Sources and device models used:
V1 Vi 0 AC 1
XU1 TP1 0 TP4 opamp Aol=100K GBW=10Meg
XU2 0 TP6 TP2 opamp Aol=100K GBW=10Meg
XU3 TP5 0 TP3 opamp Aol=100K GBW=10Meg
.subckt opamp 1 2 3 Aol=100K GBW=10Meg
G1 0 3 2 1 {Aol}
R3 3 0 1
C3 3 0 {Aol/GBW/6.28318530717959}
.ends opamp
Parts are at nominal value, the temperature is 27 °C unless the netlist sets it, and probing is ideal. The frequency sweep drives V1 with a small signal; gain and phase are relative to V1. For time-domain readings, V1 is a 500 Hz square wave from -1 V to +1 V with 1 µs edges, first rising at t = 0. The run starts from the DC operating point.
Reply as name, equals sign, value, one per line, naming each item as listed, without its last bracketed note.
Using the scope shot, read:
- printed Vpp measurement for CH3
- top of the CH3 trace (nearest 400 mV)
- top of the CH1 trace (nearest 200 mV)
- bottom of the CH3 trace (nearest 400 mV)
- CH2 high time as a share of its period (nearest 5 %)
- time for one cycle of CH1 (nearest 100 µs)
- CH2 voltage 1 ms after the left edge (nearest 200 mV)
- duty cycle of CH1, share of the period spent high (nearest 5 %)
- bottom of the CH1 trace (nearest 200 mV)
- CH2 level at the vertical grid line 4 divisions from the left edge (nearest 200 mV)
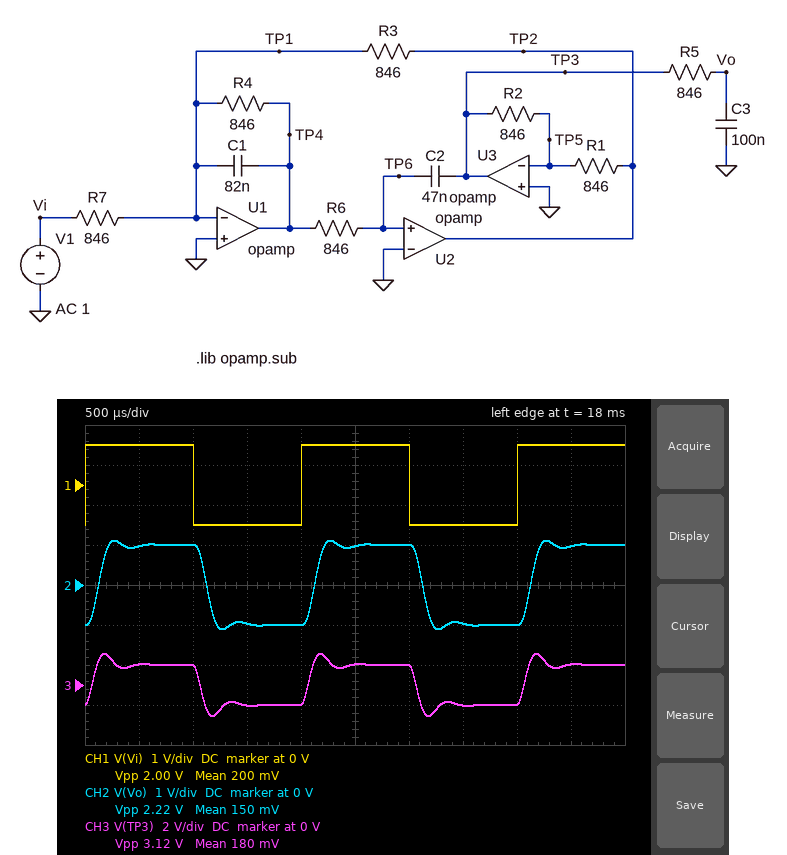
printed Vpp measurement for CH3 = 3.12 V
top of the CH3 trace = 1.6 V
top of the CH1 trace = 1.0 V
bottom of the CH3 trace = -1.6 V
CH2 high time as a share of its period = 50 %
time for one cycle of CH1 = 2.0 ms
CH2 voltage 1 ms after the left edge = 1.0 V
duty cycle of CH1, share of the period spent high = 50 %
bottom of the CH1 trace = -1.0 V
CH2 level at the vertical grid line 4 divisions from the left edge = -1.0 V
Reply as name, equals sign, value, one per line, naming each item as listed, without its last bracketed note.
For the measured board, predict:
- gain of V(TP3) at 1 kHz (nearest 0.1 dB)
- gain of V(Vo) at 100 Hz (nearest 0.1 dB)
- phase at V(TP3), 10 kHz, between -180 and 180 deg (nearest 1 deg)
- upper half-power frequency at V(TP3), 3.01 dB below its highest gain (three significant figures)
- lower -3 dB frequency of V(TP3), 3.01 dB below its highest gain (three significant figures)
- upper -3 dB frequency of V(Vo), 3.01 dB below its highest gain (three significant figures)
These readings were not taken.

gain of V(TP3) at 1 kHz = 0.7 dB
gain of V(Vo) at 100 Hz = 0 dB
phase at V(TP3), 10 kHz, between -180 and 180 deg = -166 deg
upper half-power frequency at V(TP3), 3.01 dB below its highest gain = 3.60 kHz
lower -3 dB frequency of V(TP3), 3.01 dB below its highest gain = 341 Hz
upper -3 dB frequency of V(Vo), 3.01 dB below its highest gain = 3.00 kHz
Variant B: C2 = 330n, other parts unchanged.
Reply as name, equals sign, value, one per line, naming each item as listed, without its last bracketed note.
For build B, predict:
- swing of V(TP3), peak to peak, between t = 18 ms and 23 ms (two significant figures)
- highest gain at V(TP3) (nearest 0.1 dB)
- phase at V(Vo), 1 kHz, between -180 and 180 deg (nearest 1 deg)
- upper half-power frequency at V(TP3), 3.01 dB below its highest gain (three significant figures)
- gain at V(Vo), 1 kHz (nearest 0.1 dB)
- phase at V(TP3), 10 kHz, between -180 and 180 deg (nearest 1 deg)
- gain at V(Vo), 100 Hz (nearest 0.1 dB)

swing of V(TP3), peak to peak, between t = 18 ms and 23 ms = 2.0 V
highest gain at V(TP3) = 0 dB
phase at V(Vo), 1 kHz, between -180 and 180 deg = -110 deg
upper half-power frequency at V(TP3), 3.01 dB below its highest gain = 733 Hz
gain at V(Vo), 1 kHz = -6.0 dB
phase at V(TP3), 10 kHz, between -180 and 180 deg = -167 deg
gain at V(Vo), 100 Hz = -0.1 dB
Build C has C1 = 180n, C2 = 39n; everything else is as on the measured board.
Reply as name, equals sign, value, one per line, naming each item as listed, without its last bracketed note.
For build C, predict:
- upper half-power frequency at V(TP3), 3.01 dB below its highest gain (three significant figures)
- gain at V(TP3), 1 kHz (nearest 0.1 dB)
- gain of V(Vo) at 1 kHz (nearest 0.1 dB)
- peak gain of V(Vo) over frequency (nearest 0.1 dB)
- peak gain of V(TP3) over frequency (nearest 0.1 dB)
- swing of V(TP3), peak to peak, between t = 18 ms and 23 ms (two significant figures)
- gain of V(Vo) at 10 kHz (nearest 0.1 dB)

upper half-power frequency at V(TP3), 3.01 dB below its highest gain = 2.60 kHz
gain at V(TP3), 1 kHz = 1.6 dB
gain of V(Vo) at 1 kHz = 0.6 dB
peak gain of V(Vo) over frequency = 3.4 dB
peak gain of V(TP3) over frequency = 6.9 dB
swing of V(TP3), peak to peak, between t = 18 ms and 23 ms = 3.8 V
gain of V(Vo) at 10 kHz = -40.2 dB
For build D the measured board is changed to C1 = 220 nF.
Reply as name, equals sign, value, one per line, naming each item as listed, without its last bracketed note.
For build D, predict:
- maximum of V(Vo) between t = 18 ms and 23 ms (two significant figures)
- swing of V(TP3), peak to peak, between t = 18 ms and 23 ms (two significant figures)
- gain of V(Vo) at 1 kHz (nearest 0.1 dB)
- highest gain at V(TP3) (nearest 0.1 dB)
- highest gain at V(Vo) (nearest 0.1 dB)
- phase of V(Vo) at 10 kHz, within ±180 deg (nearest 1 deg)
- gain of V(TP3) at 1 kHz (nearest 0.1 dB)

maximum of V(Vo) between t = 18 ms and 23 ms = 1.6 V
swing of V(TP3), peak to peak, between t = 18 ms and 23 ms = 3.9 V
gain of V(Vo) at 1 kHz = 1.4 dB
highest gain at V(TP3) = 6.9 dB
highest gain at V(Vo) = 4.3 dB
phase of V(Vo) at 10 kHz, within ±180 deg = 106 deg
gain of V(TP3) at 1 kHz = 2.5 dB
